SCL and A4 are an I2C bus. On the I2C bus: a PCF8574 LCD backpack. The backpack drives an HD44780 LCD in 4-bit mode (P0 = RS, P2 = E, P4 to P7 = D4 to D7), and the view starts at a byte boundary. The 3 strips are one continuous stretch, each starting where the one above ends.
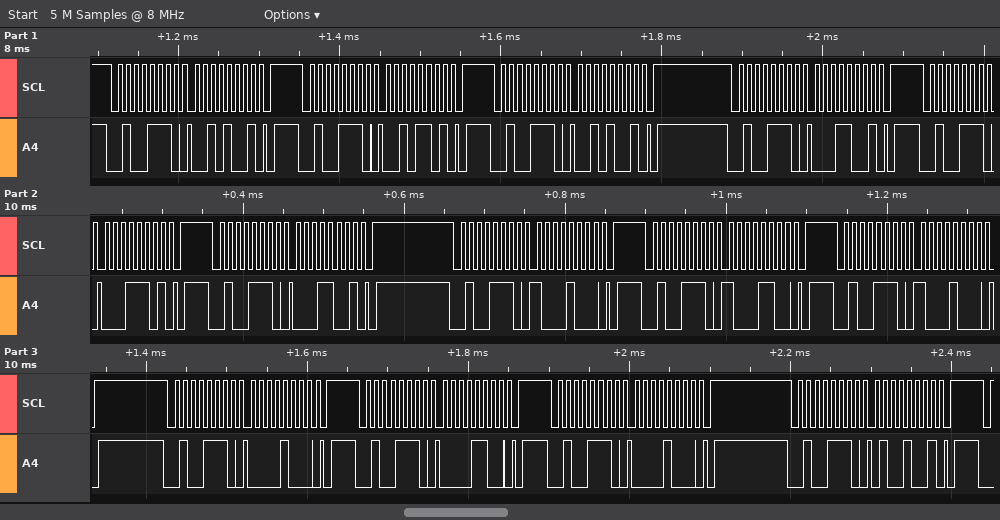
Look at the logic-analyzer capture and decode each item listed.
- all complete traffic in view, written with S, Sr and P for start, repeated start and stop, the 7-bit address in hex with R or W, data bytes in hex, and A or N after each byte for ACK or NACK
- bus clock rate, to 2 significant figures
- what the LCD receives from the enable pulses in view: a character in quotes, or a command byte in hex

S 27W A 29 A P S 27W A 2D A P S 27W A 29 A P S 27W A 19 A P S 27W A 1D A P S 27W A 19 A P S 27W A 88 A P S 27W A 8C A P S 27W A 88 A P S 27W A 08 A P S 27W A 0C A P S 27W A 08 A P S 27W A 49 A P
100 kHz
'!' 0x80
